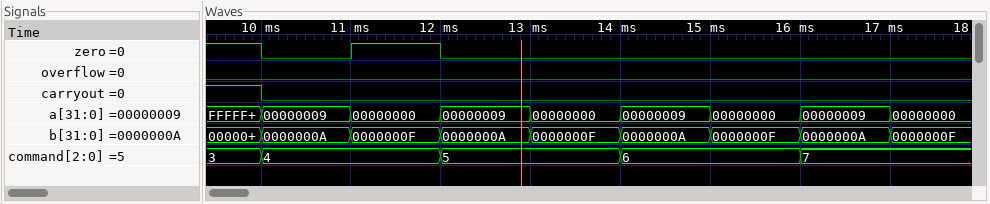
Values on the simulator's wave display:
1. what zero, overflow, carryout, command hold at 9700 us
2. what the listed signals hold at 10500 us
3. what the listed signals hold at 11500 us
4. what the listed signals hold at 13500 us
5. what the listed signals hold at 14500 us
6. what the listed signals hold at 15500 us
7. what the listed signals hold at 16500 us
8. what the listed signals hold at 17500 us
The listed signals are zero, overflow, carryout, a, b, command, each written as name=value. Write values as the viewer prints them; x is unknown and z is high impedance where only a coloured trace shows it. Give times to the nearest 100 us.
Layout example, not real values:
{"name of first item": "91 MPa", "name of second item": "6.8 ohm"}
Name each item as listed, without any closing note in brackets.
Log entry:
{"what zero, overflow, carryout, command hold at 9700 us": "zero=1, overflow=0, carryout=1, command=3", "what the listed signals hold at 10500 us": "zero=0, overflow=0, carryout=0, a=00000009, b=0000000A, command=4", "what the listed signals hold at 11500 us": "zero=1, overflow=0, carryout=0, a=00000000, b=0000000F, command=4", "what the listed signals hold at 13500 us": "zero=0, overflow=0, carryout=0, a=00000000, b=0000000F, command=5", "what the listed signals hold at 14500 us": "zero=0, overflow=0, carryout=0, a=00000009, b=0000000A, command=6", "what the listed signals hold at 15500 us": "zero=0, overflow=0, carryout=0, a=00000000, b=0000000F, command=6", "what the listed signals hold at 16500 us": "zero=0, overflow=0, carryout=0, a=00000009, b=0000000A, command=7", "what the listed signals hold at 17500 us": "zero=0, overflow=0, carryout=0, a=00000000, b=0000000F, command=7"}
